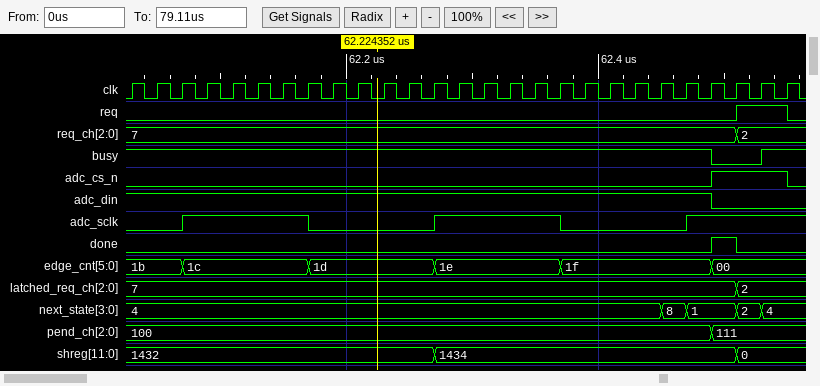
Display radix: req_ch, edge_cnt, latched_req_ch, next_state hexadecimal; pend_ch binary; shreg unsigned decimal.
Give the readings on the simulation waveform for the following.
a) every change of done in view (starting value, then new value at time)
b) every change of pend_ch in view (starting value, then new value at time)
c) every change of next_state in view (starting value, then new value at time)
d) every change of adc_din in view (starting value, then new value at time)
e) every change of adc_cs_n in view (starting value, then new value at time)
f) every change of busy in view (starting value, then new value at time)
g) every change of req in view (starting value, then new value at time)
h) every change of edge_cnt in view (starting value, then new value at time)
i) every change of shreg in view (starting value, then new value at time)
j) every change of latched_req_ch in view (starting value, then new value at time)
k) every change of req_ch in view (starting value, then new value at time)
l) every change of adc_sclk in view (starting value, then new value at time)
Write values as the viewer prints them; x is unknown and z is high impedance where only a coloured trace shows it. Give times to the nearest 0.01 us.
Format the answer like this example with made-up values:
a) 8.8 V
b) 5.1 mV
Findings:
a) 0, 1 at 62.49 us, 0 at 62.51 us
b) 100, 111 at 62.49 us
c) 4, 8 at 62.45 us, 1 at 62.47 us, 2 at 62.51 us, 4 at 62.53 us
d) 1, 0 at 62.49 us
e) 0, 1 at 62.49 us, 0 at 62.55 us
f) 1, 0 at 62.49 us, 1 at 62.53 us
g) 0, 1 at 62.51 us, 0 at 62.55 us
h) 1b, 1c at 62.07 us, 1d at 62.17 us, 1e at 62.27 us, 1f at 62.37 us, 00 at 62.49 us
i) 1432, 1434 at 62.27 us, 0 at 62.51 us
j) 7, 2 at 62.51 us
k) 7, 2 at 62.51 us
l) 0, 1 at 62.07 us, 0 at 62.17 us, 1 at 62.27 us, 0 at 62.37 us, 1 at 62.47 us
